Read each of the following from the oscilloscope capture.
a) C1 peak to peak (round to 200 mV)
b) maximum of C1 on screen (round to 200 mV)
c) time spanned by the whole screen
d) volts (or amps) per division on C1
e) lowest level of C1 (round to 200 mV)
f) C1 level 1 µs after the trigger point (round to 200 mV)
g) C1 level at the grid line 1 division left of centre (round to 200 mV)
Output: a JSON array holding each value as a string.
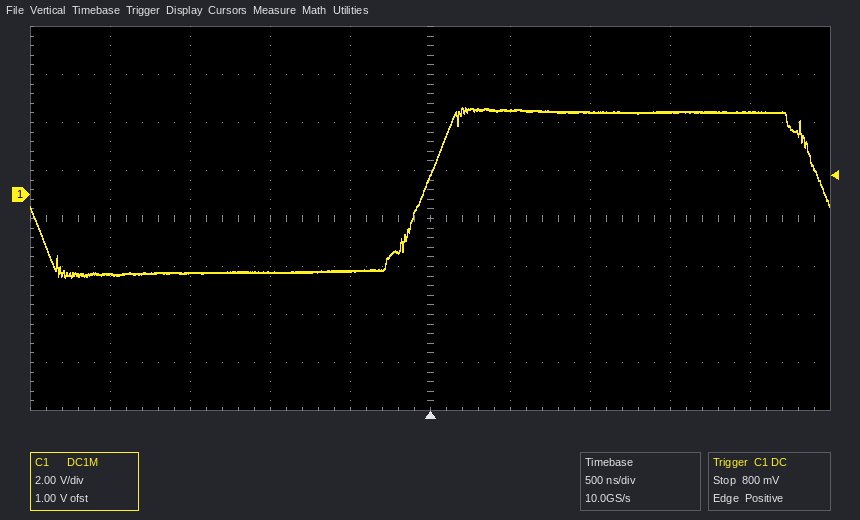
["7.0 V", "3.6 V", "5 µs", "2 V", "-3.4 V", "3.4 V", "-3.2 V"]
